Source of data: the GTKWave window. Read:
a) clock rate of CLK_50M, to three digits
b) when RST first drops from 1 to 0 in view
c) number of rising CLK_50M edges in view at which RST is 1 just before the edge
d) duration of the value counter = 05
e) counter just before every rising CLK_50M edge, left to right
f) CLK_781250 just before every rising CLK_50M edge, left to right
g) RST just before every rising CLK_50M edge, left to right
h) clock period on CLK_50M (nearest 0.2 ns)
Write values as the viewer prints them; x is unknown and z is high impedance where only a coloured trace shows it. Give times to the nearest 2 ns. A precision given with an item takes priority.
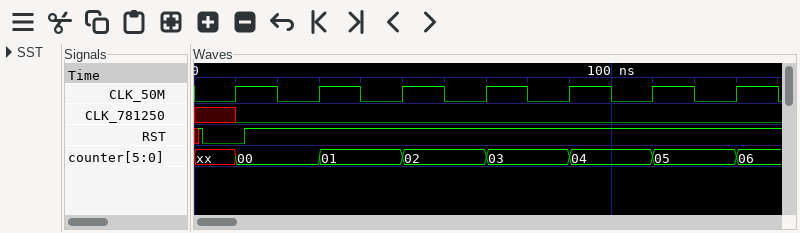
50.0 MHz
2 ns
6
20 ns
xx, 00, 01, 02, 03, 04, 05
x 0 0 0 0 0 0
0 1 1 1 1 1 1
20 ns
